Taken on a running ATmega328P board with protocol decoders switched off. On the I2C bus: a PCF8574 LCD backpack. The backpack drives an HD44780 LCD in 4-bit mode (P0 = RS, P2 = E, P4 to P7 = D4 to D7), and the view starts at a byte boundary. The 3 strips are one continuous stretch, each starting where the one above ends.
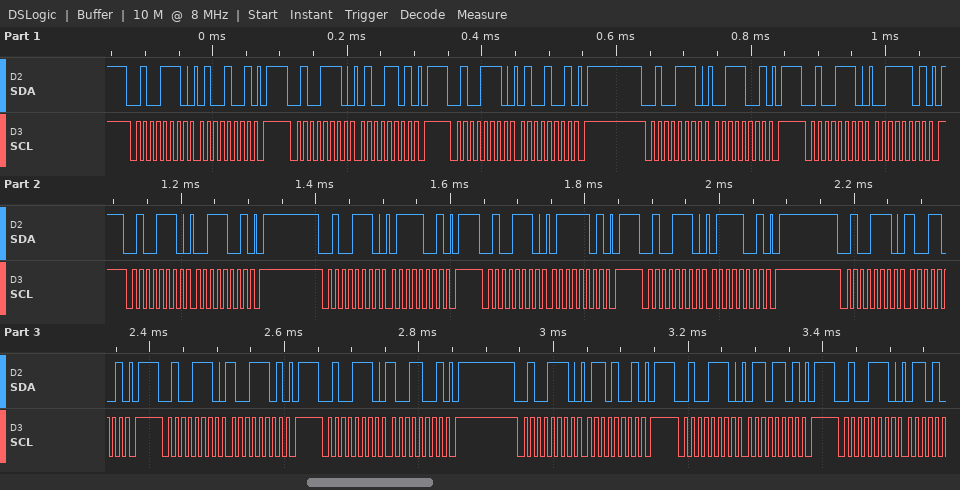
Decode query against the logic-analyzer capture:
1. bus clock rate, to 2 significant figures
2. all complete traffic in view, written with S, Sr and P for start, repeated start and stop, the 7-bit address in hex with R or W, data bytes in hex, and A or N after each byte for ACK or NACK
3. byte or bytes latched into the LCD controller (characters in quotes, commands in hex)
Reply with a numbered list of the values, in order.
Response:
1. 100 kHz
2. S 27W A 49 A P S 27W A 4D A P S 27W A 49 A P S 27W A 39 A P S 27W A 3D A P S 27W A 39 A P S 27W A 79 A P S 27W A 7D A P S 27W A 79 A P S 27W A 99 A P S 27W A 9D A P S 27W A 99 A P S 27W A 69 A P S 27W A 6D A P S 27W A
3. 'C' 'y'
